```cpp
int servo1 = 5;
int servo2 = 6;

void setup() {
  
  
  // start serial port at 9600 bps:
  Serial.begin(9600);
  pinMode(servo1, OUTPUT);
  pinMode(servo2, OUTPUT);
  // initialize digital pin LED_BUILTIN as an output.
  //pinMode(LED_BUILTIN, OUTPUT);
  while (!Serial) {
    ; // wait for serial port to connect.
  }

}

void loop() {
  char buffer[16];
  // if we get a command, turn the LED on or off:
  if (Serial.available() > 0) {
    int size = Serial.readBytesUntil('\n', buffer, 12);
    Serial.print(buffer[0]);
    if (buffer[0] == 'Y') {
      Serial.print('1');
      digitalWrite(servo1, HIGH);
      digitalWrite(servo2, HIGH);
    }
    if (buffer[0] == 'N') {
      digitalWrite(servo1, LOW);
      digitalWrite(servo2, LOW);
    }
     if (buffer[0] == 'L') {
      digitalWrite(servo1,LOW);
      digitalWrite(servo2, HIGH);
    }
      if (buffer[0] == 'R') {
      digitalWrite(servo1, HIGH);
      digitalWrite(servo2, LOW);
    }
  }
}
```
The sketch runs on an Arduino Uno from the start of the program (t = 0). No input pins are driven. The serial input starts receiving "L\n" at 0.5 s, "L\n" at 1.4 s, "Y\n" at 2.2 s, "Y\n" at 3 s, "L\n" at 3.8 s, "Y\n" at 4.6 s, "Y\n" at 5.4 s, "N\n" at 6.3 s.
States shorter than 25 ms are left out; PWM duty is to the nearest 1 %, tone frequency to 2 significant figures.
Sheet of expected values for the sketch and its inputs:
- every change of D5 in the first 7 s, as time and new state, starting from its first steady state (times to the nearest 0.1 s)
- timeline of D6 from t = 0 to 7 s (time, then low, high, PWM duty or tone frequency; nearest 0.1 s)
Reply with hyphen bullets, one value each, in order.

- 0 s low; 2.2 s high; 3.8 s low; 4.6 s high; 6.3 s low
- 0 s low; 0.5 s high; 6.3 s low
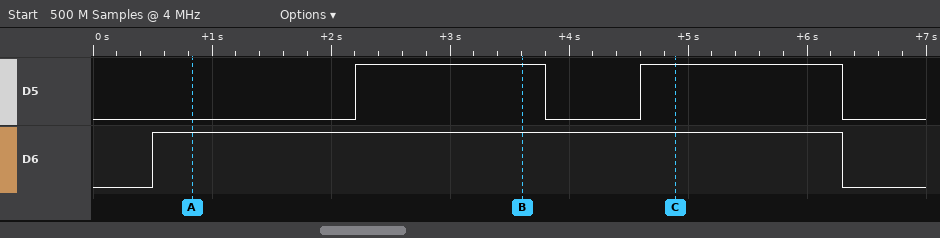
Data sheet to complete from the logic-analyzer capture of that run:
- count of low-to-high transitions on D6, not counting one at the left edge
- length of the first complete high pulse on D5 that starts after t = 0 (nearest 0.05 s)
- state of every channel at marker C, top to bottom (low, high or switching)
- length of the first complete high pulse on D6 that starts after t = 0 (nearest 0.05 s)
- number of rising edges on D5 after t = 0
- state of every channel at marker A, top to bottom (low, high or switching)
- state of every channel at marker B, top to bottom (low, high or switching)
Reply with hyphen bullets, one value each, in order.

- 1
- 1.60 s
- D5 high, D6 high
- 5.80 s
- 2
- D5 low, D6 high
- D5 high, D6 high
